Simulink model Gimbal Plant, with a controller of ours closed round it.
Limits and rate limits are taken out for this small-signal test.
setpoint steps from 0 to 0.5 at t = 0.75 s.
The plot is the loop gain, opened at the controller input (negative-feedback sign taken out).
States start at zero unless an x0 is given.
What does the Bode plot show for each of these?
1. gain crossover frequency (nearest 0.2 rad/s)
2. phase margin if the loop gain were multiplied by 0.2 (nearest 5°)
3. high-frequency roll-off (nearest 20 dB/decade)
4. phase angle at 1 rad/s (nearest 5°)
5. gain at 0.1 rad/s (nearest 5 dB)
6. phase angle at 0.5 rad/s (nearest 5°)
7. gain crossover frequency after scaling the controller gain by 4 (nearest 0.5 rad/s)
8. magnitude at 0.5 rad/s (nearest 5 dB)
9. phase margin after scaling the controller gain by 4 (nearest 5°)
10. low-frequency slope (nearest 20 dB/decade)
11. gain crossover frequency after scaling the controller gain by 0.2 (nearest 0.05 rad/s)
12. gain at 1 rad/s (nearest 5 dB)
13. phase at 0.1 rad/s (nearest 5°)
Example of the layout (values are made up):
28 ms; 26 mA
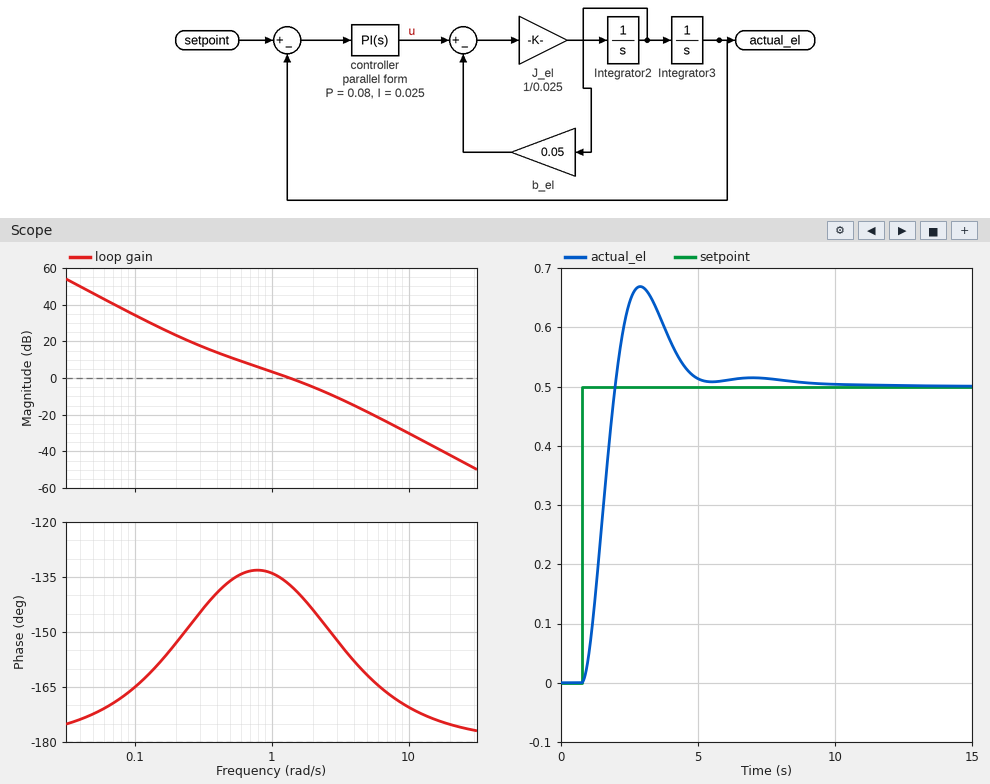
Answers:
1.4 rad/s; 40°; -40 dB/decade; -135°; 35 dB; -135°; 3.5 rad/s; 10 dB; 25°; -40 dB/decade; 0.40 rad/s; 5 dB; -165°
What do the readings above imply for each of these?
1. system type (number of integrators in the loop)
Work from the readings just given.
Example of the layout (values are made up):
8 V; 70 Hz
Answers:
2
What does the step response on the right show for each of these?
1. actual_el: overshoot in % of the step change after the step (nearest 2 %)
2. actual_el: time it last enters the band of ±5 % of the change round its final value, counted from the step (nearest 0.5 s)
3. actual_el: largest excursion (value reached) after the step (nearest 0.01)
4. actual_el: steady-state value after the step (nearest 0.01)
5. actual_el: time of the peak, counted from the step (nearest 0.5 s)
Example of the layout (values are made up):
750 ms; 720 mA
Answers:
34 %; 4.0 s; 0.67; 0.50; 2.0 s
